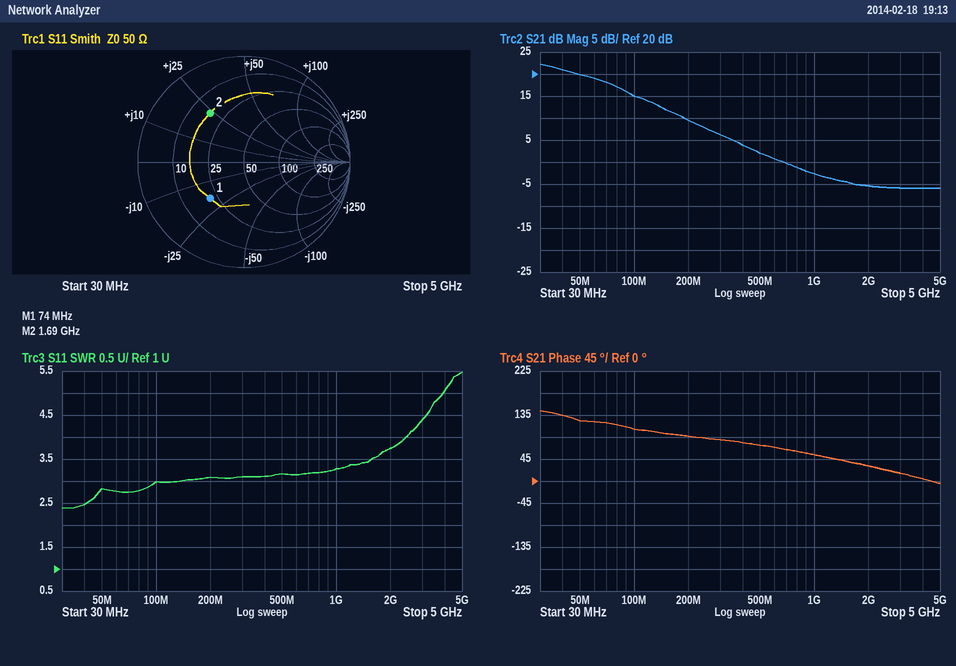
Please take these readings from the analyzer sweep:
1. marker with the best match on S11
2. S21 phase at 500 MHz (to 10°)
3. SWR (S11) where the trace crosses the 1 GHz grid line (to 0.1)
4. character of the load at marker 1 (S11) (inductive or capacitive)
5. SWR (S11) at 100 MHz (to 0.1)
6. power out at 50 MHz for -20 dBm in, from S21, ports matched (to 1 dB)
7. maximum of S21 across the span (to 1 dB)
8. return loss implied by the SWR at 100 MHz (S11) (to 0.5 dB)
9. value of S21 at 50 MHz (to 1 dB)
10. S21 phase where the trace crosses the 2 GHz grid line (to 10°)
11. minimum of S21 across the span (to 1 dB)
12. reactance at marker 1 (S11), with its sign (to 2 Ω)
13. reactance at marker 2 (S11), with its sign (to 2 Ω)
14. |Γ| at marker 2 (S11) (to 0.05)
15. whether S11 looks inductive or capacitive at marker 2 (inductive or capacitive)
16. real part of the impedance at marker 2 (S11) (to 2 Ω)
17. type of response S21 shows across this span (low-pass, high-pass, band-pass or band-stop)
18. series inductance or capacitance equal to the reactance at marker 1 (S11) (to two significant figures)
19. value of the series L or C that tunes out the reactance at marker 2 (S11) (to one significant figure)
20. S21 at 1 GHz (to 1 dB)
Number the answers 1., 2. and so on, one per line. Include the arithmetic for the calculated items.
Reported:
1. marker 1
2. 70°
3. 3.3
4. capacitive
5. 3.0
6. -20 dBm + (20 dB) = 0 dBm
7. 22 dB
8. −20 log10((3 − 1)/(3 + 1)) ≈ 6.0 dB
9. 20 dB
10. 30°
11. -6 dB
12. -18 Ω
13. +24 Ω
14. 0.55
15. inductive
16. 18 Ω
17. low-pass
18. C = 1/(2π × 74 MHz × 18 Ω) ≈ 119 pF, so 120 pF to two significant figures
19. C = 1/(2π × 1.69 GHz × 24 Ω) ≈ 4 pF
20. -3 dB
